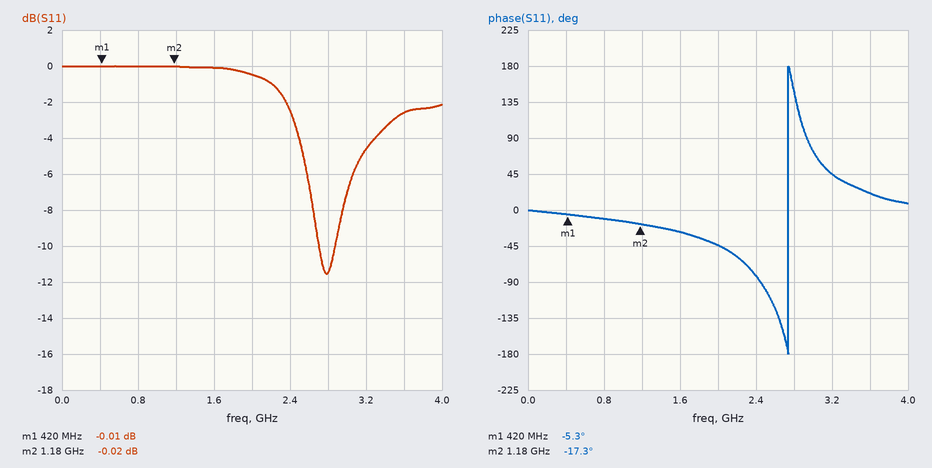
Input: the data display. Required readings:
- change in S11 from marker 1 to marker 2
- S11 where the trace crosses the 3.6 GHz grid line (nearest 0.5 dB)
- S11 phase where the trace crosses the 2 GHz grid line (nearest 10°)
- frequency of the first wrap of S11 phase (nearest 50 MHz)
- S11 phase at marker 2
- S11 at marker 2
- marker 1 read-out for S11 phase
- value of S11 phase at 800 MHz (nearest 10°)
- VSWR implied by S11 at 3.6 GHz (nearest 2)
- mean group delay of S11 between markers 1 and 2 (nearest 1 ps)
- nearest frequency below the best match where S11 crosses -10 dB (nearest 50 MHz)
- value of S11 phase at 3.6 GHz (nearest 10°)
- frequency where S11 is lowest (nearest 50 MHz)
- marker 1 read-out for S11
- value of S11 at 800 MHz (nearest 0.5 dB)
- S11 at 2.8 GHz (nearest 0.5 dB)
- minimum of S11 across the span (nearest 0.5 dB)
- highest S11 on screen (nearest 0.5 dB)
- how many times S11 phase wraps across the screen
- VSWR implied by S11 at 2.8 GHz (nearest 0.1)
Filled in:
-0.01 dB
-2.5 dB
-40°
2.75 GHz
-17.3°
-0.02 dB
-5.3°
-10°
6
44 ps
2.70 GHz
20°
2.80 GHz
-0.01 dB
0.0 dB
-11.5 dB
-11.5 dB
0.0 dB
1
1.7
